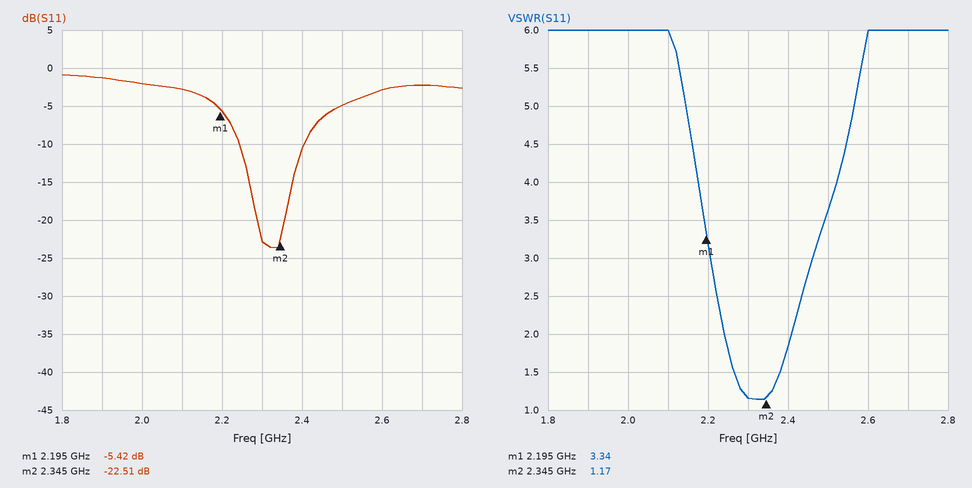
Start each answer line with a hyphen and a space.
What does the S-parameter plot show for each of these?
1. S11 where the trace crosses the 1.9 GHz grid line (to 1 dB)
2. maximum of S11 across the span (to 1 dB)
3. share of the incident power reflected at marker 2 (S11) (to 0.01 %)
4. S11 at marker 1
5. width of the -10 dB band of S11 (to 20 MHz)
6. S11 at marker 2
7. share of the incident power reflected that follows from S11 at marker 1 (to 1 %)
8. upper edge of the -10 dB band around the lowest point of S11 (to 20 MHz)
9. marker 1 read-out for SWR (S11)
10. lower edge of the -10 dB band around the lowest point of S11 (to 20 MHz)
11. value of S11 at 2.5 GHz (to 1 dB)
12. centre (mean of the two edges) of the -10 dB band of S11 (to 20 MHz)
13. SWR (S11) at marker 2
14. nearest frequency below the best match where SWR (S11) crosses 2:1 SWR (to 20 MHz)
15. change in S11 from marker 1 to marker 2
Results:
- -1 dB
- -1 dB
- 0.56 %
- -5.42 dB
- 160 MHz
- -22.51 dB
- 29 %
- 2.40 GHz
- 3.34
- 2.24 GHz
- -5 dB
- 2.32 GHz
- 1.17
- 2.24 GHz
- -17.09 dB
